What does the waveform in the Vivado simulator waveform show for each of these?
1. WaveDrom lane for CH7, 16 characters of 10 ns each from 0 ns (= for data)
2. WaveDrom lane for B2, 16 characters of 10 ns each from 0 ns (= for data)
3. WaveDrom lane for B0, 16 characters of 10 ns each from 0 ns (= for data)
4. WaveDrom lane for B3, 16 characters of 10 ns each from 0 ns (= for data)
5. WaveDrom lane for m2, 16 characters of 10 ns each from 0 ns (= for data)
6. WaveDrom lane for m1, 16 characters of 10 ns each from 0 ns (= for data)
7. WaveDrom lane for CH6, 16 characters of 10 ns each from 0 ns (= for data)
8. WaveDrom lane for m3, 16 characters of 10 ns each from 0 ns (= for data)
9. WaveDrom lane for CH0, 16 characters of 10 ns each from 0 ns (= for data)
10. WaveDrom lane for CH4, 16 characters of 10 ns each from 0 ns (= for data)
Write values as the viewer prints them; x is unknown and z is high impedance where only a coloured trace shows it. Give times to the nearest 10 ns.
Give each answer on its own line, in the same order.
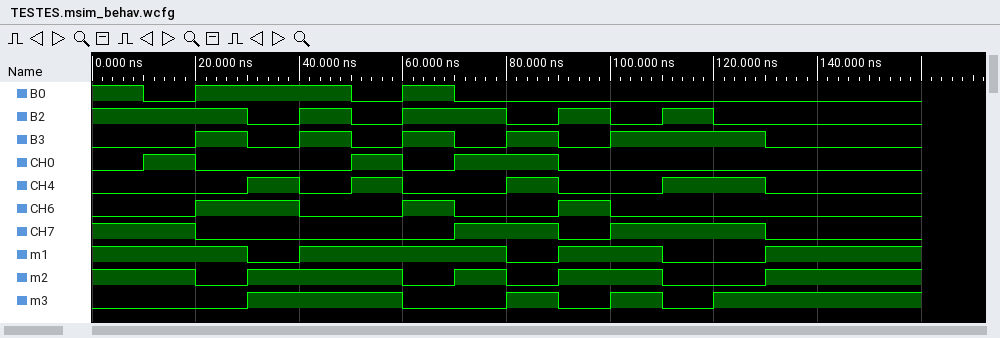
{name: 'CH7', wave: '1.0....1.01..0..'}
{name: 'B2', wave: '1..0101.01010...'}
{name: 'B0', wave: '101..010........'}
{name: 'B3', wave: '0.101010101..0..'}
{name: 'm2', wave: '1.01..0101.0.1..'}
{name: 'm1', wave: '1..01...01.0.1..'}
{name: 'CH6', wave: '0.1.0.10.10.....'}
{name: 'm3', wave: '0..1..0.10101...'}
{name: 'CH0', wave: '010..101.0......'}
{name: 'CH4', wave: '0..1010.10.1.0..'}
